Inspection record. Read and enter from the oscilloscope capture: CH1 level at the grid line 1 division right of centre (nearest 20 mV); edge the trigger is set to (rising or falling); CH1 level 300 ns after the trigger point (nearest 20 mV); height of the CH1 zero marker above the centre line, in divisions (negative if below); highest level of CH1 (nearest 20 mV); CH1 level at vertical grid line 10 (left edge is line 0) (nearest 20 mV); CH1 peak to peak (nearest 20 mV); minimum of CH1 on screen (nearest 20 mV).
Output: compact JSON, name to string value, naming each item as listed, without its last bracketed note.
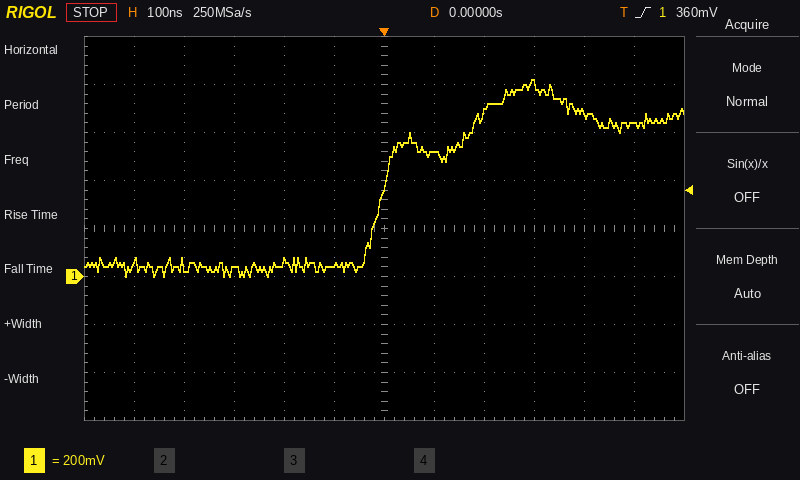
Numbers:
{"CH1 level at the grid line 1 division right of centre": "520 mV", "edge the trigger is set to": "rising", "CH1 level 300 ns after the trigger point": "800 mV", "height of the CH1 zero marker above the centre line, in divisions": "-1.0 div", "highest level of CH1": "820 mV", "CH1 level at vertical grid line 10 (left edge is line 0)": "680 mV", "CH1 peak to peak": "820 mV", "minimum of CH1 on screen": "0 mV"}
